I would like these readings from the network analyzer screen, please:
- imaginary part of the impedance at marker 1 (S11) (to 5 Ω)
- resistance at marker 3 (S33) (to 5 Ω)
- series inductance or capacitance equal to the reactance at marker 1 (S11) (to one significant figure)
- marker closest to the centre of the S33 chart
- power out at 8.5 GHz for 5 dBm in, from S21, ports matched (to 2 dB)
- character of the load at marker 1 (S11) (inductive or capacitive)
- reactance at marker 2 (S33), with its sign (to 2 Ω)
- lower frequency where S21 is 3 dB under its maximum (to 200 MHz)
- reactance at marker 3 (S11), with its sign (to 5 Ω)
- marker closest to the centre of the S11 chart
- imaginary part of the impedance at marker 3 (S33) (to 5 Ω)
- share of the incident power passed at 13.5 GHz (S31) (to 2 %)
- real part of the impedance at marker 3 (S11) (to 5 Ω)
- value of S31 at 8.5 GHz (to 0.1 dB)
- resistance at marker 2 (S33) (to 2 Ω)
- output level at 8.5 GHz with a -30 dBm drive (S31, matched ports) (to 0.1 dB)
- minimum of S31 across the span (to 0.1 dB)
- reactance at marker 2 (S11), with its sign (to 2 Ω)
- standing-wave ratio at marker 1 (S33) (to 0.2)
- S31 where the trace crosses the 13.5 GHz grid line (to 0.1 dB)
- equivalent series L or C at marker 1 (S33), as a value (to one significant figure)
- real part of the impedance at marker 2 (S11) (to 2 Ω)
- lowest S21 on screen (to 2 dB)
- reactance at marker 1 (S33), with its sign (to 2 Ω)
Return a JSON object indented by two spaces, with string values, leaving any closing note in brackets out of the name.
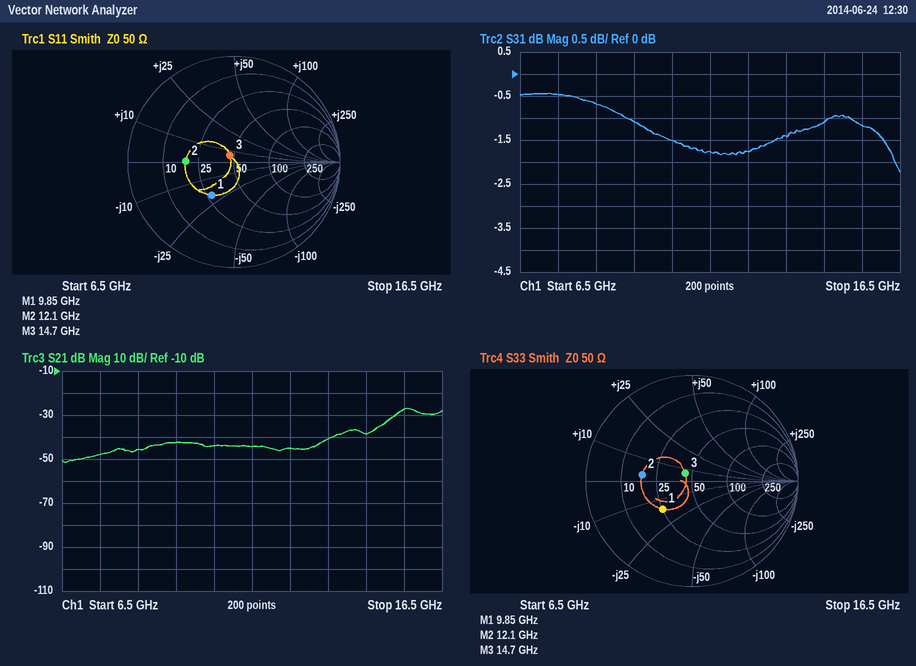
{
  "imaginary part of the impedance at marker 1 (S11)": "-20 Ω",
  "resistance at marker 3 (S33)": "45 Ω",
  "series inductance or capacitance equal to the reactance at marker 1 (S11)": "800 fF",
  "marker closest to the centre of the S33 chart": "marker 3",
  "power out at 8.5 GHz for 5 dBm in, from S21, ports matched": "-40 dBm",
  "character of the load at marker 1 (S11)": "capacitive",
  "reactance at marker 2 (S33), with its sign": "+2 Ω",
  "lower frequency where S21 is 3 dB under its maximum": "15.2 GHz",
  "reactance at marker 3 (S11), with its sign": "+5 Ω",
  "marker closest to the centre of the S11 chart": "marker 3",
  "imaginary part of the impedance at marker 3 (S33)": "+5 Ω",
  "share of the incident power passed at 13.5 GHz (S31)": "72 %",
  "real part of the impedance at marker 3 (S11)": "45 Ω",
  "value of S31 at 8.5 GHz": "-0.7 dB",
  "resistance at marker 2 (S33)": "18 Ω",
  "output level at 8.5 GHz with a -30 dBm drive (S31, matched ports)": "-30.7 dBm",
  "minimum of S31 across the span": "-2.2 dB",
  "reactance at marker 2 (S11), with its sign": "0 Ω",
  "standing-wave ratio at marker 1 (S33)": "2.2",
  "S31 where the trace crosses the 13.5 GHz grid line": "-1.4 dB",
  "equivalent series L or C at marker 1 (S33), as a value": "1 pF",
  "real part of the impedance at marker 2 (S11)": "18 Ω",
  "lowest S21 on screen": "-52 dB",
  "reactance at marker 1 (S33), with its sign": "-16 Ω"
}
